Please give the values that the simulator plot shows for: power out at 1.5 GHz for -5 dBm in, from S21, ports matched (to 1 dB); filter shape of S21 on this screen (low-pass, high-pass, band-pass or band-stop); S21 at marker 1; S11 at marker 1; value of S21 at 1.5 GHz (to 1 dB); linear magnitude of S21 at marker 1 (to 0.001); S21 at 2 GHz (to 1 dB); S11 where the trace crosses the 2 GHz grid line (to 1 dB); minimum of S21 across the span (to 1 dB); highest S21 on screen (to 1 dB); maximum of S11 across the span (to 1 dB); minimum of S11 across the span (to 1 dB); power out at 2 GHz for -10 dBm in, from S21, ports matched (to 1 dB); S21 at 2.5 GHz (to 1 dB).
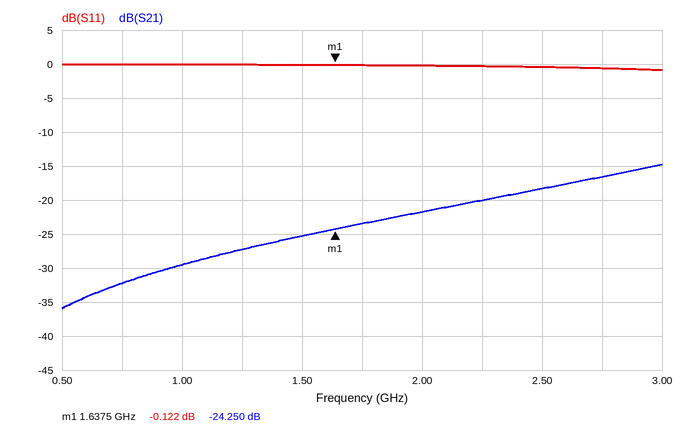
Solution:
-30 dBm
high-pass
-24.250 dB
-0.122 dB
-25 dB
0.061
-22 dB
0 dB
-36 dB
-15 dB
0 dB
-1 dB
-32 dBm
-18 dB
